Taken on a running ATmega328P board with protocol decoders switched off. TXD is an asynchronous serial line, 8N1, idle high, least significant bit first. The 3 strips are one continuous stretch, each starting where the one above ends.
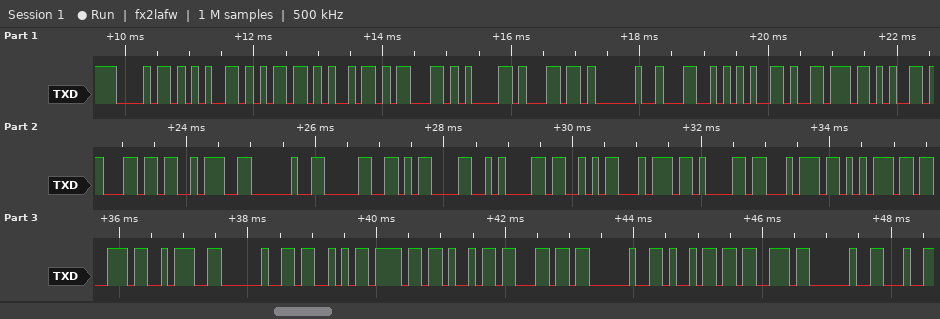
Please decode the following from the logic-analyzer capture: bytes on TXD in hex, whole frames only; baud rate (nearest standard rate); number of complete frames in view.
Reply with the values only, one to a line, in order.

0x68 0x65 0x6D 0x69 0x63 0x61 0x6C 0x20 0x4C 0x65 0x76 0x65 0x6C 0x3A 0x20 0x30 0x0D 0x0A 0x53 0x74 0x61 0x74 0x75 0x73 0x3A 0x20 0x53 0x6F 0x69 0x6C 0x20 0x69 0x73 0x20
9600 baud
34
